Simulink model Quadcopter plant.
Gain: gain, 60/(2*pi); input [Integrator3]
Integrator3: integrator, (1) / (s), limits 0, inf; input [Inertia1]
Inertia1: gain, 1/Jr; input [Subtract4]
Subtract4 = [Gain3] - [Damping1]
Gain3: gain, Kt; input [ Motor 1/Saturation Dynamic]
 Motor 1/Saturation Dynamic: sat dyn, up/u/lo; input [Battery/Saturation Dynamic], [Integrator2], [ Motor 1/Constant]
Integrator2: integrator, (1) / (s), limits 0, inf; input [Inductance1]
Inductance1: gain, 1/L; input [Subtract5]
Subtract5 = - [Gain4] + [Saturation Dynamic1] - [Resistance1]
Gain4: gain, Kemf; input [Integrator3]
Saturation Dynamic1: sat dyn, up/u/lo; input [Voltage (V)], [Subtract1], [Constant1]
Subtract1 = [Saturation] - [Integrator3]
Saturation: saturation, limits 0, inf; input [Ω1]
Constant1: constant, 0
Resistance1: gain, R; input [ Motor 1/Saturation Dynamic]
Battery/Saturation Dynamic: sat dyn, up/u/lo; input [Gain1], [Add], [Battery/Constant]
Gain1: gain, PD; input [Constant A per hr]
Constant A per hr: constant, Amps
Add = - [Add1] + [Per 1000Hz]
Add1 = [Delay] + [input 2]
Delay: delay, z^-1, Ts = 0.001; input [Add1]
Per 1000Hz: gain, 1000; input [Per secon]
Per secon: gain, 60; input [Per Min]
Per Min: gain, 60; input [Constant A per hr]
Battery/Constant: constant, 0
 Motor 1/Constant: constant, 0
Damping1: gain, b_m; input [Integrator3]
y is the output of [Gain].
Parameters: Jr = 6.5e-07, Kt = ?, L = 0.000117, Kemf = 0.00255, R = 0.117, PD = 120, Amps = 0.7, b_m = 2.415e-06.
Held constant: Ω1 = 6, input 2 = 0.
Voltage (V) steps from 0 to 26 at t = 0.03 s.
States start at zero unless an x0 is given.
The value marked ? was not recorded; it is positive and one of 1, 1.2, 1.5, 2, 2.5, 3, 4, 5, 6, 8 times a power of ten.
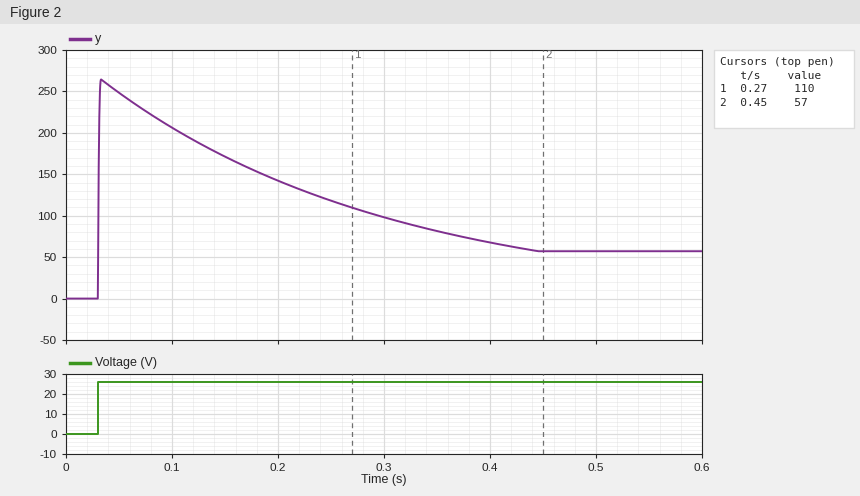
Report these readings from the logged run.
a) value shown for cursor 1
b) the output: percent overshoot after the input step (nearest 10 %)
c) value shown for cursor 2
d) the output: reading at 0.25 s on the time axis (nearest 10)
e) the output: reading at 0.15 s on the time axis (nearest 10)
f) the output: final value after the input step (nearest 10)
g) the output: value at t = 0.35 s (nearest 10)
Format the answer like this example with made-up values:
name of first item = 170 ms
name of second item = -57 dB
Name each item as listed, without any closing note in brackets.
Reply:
value shown for cursor 1 = 110
the output: percent overshoot after the input step = 360 %
value shown for cursor 2 = 57
the output: reading at 0.25 s on the time axis = 120
the output: reading at 0.15 s on the time axis = 170
the output: final value after the input step = 60
the output: value at t = 0.35 s = 80
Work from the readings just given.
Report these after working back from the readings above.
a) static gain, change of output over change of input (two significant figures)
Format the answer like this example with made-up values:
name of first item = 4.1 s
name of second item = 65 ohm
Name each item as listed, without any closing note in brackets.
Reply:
static gain, change of output over change of input = 2.3
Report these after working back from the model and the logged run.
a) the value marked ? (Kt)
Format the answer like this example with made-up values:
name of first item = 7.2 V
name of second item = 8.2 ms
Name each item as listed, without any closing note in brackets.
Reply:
the value marked ? = 0.002
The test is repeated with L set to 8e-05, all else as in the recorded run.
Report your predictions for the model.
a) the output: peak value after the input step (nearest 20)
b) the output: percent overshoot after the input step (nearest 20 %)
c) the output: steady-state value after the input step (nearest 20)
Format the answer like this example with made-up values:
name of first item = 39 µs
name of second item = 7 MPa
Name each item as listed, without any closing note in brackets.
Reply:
the output: peak value after the input step = 220
the output: percent overshoot after the input step = 300 %
the output: steady-state value after the input step = 60
